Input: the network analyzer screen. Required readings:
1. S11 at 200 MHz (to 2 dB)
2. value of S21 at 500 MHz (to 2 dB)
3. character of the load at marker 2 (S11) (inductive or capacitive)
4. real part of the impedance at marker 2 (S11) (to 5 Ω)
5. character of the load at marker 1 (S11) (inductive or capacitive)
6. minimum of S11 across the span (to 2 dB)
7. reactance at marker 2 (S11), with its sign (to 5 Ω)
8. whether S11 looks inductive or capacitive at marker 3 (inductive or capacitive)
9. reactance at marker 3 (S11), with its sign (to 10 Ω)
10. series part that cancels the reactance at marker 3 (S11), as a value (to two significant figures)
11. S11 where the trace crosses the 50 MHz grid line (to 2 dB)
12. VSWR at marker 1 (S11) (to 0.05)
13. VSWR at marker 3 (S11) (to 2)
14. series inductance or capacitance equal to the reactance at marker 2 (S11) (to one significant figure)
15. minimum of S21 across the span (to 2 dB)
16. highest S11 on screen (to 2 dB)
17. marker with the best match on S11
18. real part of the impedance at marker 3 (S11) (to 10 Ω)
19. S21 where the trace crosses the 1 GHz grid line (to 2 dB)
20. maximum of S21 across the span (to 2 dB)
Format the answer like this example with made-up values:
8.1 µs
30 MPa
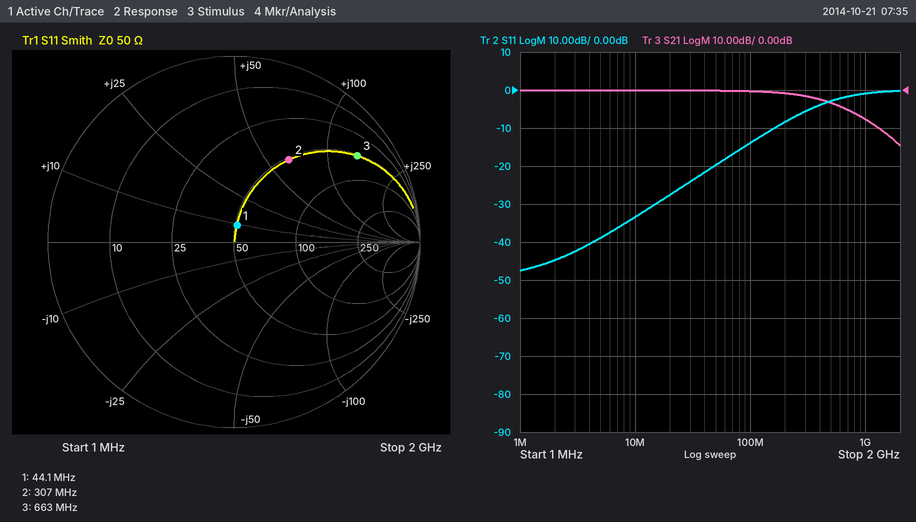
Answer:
-8 dB
-4 dB
inductive
50 Ω
inductive
-48 dB
+65 Ω
inductive
+140 Ω
1.7 pF
-20 dB
1.20
10
30 nH
-14 dB
0 dB
marker 1
50 Ω
-8 dB
0 dB
